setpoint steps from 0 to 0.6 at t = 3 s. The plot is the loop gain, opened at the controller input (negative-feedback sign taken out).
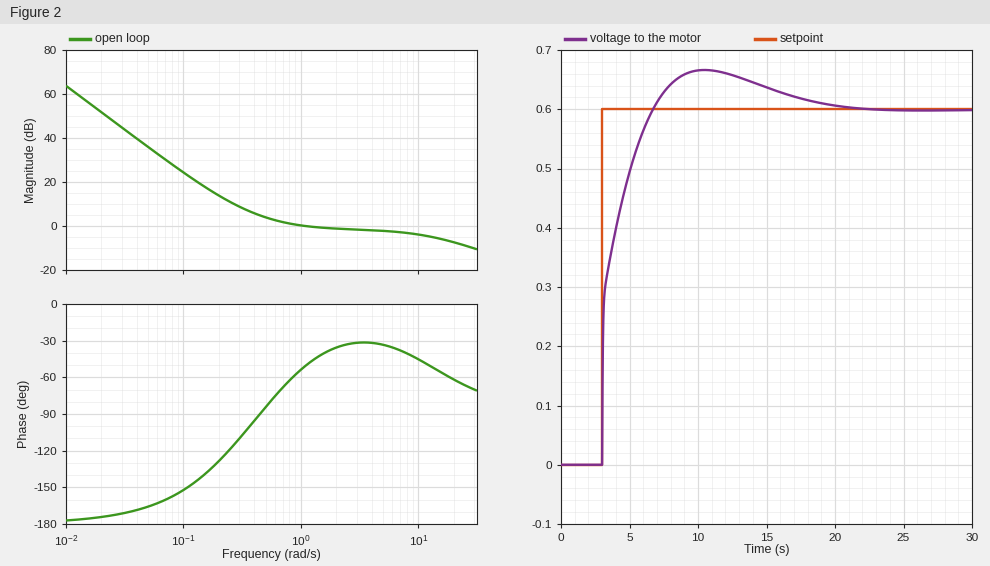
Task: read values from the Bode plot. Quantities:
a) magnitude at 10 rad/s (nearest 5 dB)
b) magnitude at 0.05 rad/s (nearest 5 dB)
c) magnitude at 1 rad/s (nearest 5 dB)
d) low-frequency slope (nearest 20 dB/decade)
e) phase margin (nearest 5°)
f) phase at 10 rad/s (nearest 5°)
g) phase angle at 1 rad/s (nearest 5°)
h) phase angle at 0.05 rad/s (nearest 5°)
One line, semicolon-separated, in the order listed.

-5 dB; 35 dB; 0 dB; -40 dB/decade; 130°; -45°; -55°; -165°
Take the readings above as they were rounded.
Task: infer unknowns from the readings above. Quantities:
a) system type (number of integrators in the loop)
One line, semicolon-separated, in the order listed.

2
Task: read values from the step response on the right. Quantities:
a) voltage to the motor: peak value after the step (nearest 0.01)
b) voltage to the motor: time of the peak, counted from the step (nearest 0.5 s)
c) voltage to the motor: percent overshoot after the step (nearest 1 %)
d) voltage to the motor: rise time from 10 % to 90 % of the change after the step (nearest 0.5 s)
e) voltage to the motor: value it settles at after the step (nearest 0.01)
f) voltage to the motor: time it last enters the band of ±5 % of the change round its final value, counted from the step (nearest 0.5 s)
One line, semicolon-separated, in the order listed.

0.67; 7.5 s; 11 %; 2.5 s; 0.60; 13.0 s
